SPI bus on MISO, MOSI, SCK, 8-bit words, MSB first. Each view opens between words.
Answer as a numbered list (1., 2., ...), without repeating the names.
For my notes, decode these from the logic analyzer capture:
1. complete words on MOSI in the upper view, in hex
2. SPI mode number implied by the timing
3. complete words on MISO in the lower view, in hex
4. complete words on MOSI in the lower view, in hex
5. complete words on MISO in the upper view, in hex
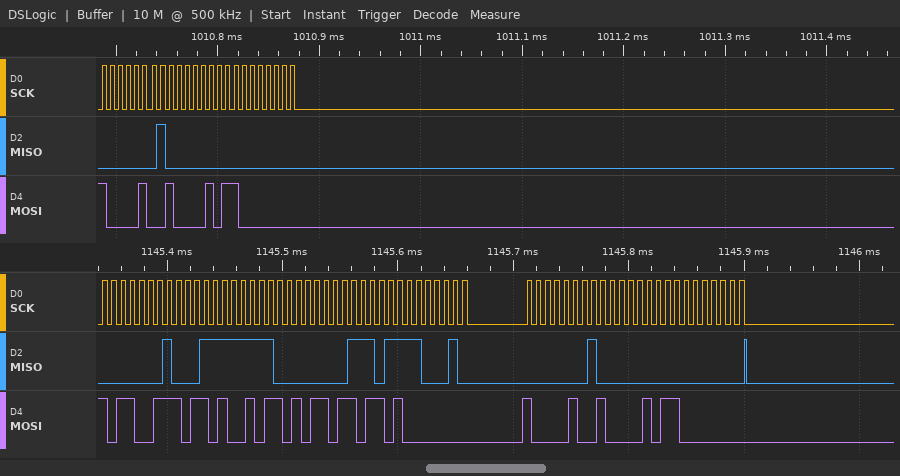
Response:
1. 84, 85, 80
2. 0
3. 01, 1F, E0, 1D, E2, 01, 00, 00
4. B3, B4, B5, B6, 80, 84, 85, 80
5. 01, 00, 00
